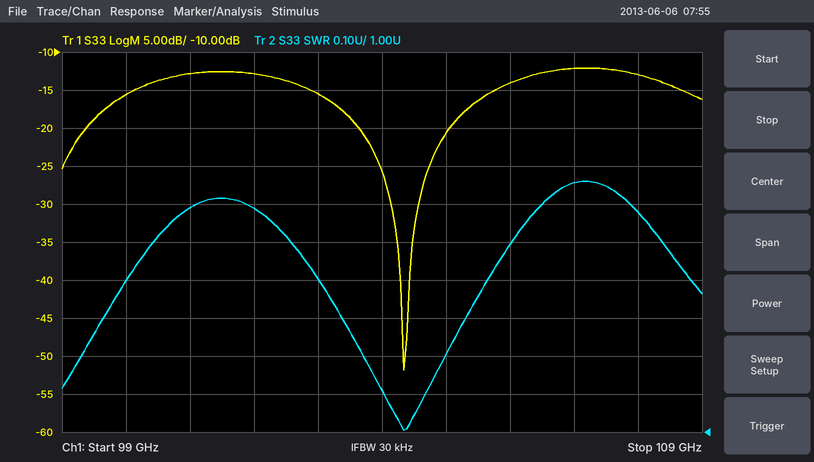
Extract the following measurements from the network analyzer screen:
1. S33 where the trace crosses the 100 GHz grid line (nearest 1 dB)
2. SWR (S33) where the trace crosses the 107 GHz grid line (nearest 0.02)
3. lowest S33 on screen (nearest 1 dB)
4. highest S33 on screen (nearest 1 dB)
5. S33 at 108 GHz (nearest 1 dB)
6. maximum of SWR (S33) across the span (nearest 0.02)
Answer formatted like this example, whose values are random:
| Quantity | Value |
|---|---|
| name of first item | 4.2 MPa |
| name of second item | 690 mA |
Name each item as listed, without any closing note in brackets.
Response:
| Quantity | Value |
|---|---|
| S33 where the trace crosses the 100 GHz grid line | -16 dB |
| SWR (S33) where the trace crosses the 107 GHz grid line | 1.66 |
| lowest S33 on screen | -52 dB |
| highest S33 on screen | -12 dB |
| S33 at 108 GHz | -13 dB |
| maximum of SWR (S33) across the span | 1.66 |
